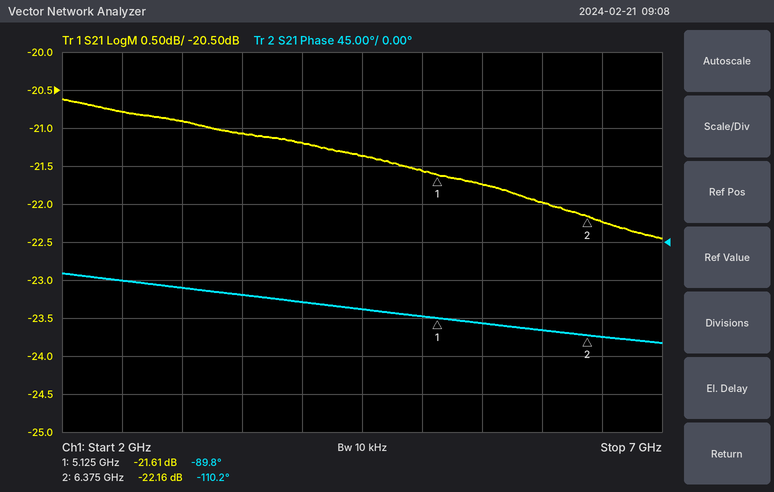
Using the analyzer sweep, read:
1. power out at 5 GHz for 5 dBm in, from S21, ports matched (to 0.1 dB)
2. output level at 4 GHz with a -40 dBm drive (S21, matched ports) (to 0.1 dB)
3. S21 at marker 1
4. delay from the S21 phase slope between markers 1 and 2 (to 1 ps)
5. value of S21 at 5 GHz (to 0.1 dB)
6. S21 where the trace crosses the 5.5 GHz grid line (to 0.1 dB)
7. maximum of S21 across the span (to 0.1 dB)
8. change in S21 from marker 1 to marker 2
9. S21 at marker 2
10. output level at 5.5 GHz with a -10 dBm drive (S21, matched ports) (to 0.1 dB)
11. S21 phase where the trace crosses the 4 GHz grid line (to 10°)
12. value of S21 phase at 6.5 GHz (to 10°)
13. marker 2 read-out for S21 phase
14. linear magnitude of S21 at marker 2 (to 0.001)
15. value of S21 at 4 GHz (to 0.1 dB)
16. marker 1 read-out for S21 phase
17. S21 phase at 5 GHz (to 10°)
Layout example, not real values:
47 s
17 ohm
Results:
-16.6 dBm
-61.2 dBm
-21.61 dB
45 ps
-21.6 dB
-21.7 dB
-20.6 dB
-0.55 dB
-22.16 dB
-31.7 dBm
-70°
-110°
-110.2°
0.078
-21.2 dB
-89.8°
-90°
